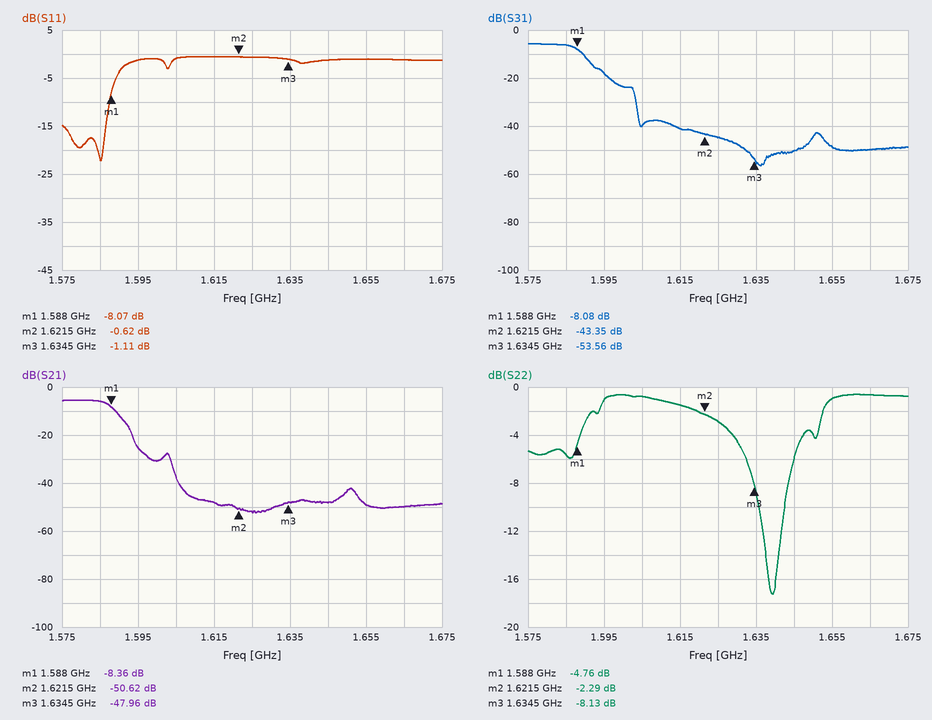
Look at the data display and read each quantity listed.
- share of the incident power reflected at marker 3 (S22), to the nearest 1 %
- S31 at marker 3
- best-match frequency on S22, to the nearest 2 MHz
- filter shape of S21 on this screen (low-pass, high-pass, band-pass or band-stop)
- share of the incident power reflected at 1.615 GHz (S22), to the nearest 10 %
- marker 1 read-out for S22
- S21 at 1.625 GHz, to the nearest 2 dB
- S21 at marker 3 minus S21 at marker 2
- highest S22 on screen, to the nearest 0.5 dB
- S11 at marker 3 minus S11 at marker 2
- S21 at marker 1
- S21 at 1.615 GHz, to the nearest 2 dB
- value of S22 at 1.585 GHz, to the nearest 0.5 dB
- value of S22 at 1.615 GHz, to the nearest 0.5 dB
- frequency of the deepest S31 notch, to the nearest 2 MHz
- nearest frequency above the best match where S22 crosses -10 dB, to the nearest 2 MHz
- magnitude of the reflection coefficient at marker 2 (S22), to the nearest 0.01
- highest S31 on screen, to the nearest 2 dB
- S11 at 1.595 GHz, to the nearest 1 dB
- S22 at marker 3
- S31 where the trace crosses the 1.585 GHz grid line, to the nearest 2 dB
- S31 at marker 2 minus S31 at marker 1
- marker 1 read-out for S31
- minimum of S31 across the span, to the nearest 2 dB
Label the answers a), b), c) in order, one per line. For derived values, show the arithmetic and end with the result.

a) 10^(-8.13/10) ≈ 15 %
b) -53.56 dB
c) 1.640 GHz
d) low-pass
e) 10^(-1.5/10) ≈ 70.8 %, so 70 % to the nearest 10 %
f) -4.76 dB
g) -52 dB
h) -47.96 − (-50.62) = 2.66 dB
i) -0.5 dB
j) -1.11 − (-0.62) = -0.49 dB
k) -8.36 dB
l) -48 dB
m) -5.5 dB
n) -1.5 dB
o) 1.636 GHz
p) 1.642 GHz
q) 10^(-2.29/20) ≈ 0.77
r) -6 dB
s) -1 dB
t) -8.13 dB
u) -6 dB
v) -43.35 − (-8.08) = -35.27 dB
w) -8.08 dB
x) -56 dB
